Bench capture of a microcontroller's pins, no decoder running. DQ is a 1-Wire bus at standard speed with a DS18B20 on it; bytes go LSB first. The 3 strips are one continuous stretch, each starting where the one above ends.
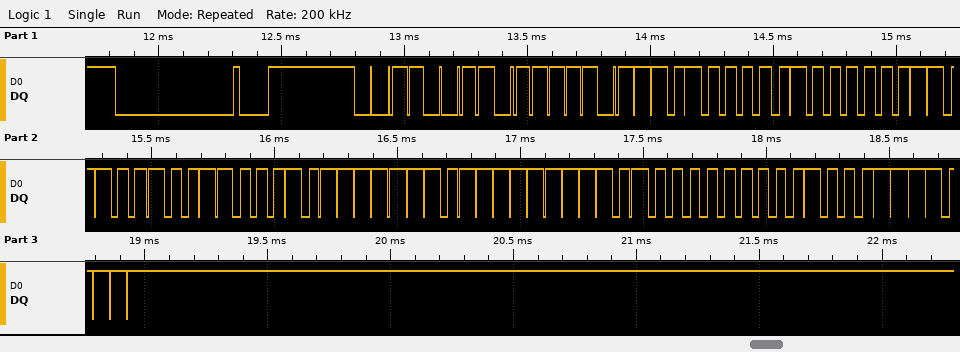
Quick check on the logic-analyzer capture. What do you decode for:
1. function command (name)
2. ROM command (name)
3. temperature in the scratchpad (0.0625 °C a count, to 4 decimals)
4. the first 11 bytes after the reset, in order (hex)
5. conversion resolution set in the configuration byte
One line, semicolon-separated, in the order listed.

Read Scratchpad; Skip ROM; 32.6875 °C; CC BE 0B 02 4B 46 7F FF 05 10 EF; 12 bits
